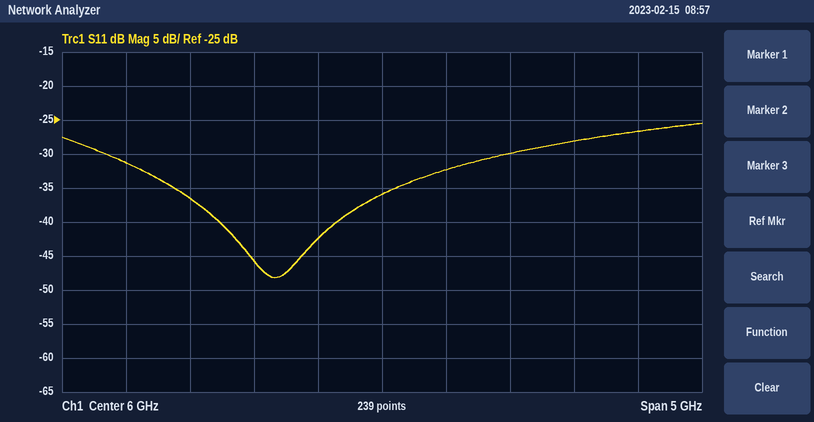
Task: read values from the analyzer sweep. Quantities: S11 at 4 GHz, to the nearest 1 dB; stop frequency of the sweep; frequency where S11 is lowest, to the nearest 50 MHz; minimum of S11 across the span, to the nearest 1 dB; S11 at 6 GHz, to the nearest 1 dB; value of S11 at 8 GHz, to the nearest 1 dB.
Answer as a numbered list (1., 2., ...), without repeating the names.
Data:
1. -31 dB
2. 8.5 GHz
3. 5.15 GHz
4. -48 dB
5. -36 dB
6. -27 dB
